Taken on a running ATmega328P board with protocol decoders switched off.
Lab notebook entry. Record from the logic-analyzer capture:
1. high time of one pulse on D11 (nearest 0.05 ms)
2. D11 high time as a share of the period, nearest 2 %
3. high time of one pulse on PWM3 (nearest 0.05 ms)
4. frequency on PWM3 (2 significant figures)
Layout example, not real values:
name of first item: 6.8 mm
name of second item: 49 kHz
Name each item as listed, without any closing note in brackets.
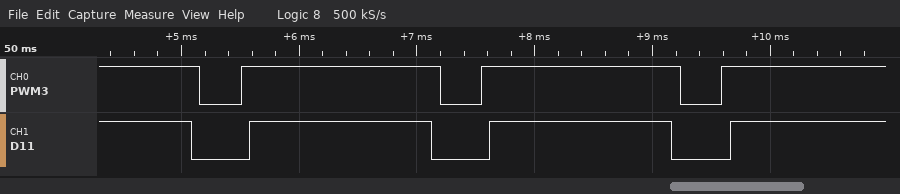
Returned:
high time of one pulse on D11: 1.55 ms
D11 high time as a share of the period, nearest 2 %: 76 %
high time of one pulse on PWM3: 1.70 ms
frequency on PWM3: 490 Hz
